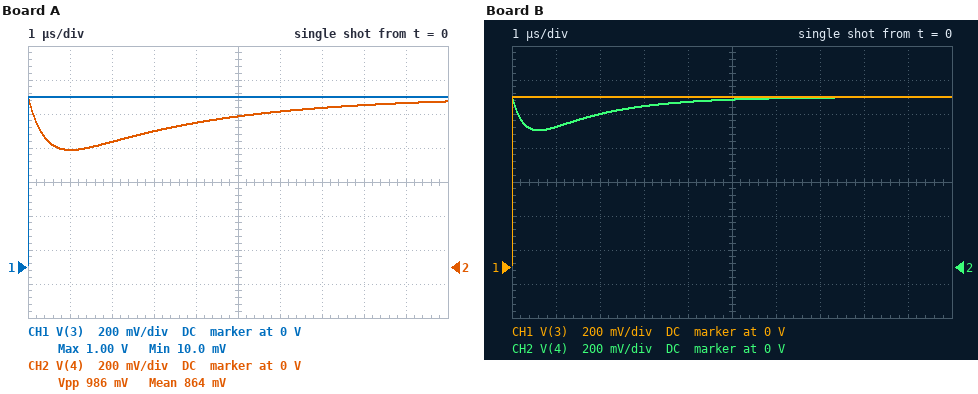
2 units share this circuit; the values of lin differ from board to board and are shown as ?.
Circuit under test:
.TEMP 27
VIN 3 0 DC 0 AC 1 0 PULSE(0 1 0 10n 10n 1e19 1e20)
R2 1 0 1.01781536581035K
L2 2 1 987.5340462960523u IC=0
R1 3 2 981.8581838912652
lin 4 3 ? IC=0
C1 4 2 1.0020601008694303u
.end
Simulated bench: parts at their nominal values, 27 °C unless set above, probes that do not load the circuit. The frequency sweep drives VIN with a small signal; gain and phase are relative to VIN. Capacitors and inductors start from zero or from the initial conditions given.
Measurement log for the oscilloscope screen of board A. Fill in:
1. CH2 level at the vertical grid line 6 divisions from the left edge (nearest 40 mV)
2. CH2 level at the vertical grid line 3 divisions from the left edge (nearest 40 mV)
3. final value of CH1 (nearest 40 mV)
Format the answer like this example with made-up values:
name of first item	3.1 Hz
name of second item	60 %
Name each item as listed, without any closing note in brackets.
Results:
CH2 level at the vertical grid line 6 divisions from the left edge	920 mV
CH2 level at the vertical grid line 3 divisions from the left edge	800 mV
final value of CH1	1.00 V
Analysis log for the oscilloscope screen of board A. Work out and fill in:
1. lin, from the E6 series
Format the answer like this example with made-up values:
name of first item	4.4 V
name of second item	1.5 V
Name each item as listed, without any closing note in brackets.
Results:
lin, from the E6 series	1.5 mH
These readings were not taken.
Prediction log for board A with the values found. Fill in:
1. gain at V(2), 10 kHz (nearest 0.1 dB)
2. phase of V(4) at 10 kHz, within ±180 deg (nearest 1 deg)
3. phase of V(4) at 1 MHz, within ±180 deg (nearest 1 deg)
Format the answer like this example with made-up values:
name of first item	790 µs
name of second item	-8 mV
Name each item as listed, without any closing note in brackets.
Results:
gain at V(2), 10 kHz	-0.1 dB
phase of V(4) at 10 kHz, within ±180 deg	-5 deg
phase of V(4) at 1 MHz, within ±180 deg	8 deg
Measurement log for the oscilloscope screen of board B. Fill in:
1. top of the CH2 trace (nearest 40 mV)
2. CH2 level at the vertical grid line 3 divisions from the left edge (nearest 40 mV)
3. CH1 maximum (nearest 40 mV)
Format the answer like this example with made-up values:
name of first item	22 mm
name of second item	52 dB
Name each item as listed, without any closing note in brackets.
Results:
top of the CH2 trace	1.00 V
CH2 level at the vertical grid line 3 divisions from the left edge	960 mV
CH1 maximum	1.00 V
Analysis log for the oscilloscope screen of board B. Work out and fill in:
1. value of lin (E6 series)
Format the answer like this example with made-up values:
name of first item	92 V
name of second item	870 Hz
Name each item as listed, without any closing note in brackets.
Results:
value of lin	470 µH
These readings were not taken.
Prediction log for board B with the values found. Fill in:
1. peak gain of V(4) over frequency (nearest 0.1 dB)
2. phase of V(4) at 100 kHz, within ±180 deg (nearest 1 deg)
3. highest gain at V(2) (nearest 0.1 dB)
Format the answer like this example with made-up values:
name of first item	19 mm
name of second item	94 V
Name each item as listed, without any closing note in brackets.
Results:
peak gain of V(4) over frequency	0 dB
phase of V(4) at 100 kHz, within ±180 deg	-8 deg
highest gain at V(2)	0 dB
